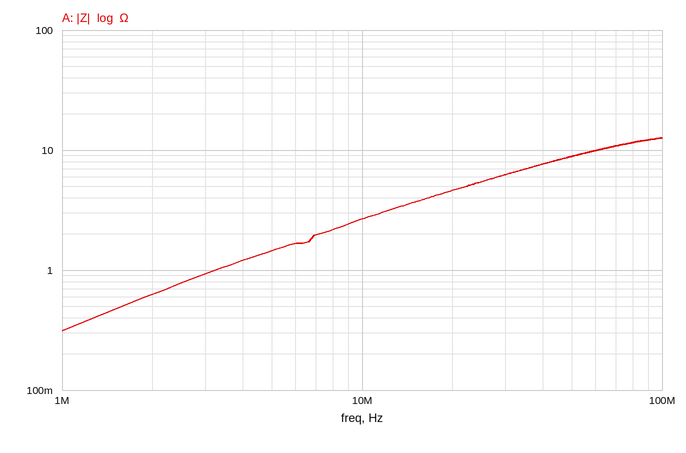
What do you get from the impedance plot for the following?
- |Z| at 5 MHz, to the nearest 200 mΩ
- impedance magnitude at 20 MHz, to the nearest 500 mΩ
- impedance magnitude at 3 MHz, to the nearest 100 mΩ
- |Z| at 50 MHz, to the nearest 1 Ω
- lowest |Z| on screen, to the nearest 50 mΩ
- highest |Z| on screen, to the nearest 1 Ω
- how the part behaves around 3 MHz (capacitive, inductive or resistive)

1.4 Ω
4.5 Ω
900 mΩ
9 Ω
300 mΩ
13 Ω
inductive
